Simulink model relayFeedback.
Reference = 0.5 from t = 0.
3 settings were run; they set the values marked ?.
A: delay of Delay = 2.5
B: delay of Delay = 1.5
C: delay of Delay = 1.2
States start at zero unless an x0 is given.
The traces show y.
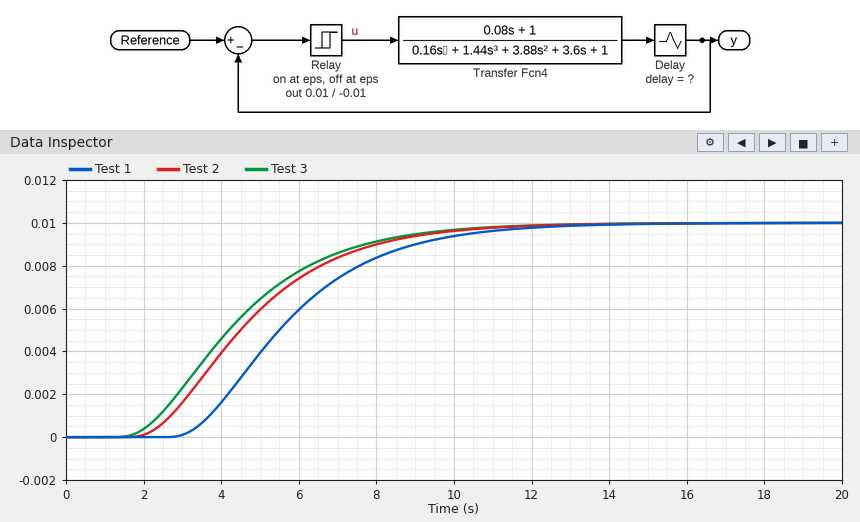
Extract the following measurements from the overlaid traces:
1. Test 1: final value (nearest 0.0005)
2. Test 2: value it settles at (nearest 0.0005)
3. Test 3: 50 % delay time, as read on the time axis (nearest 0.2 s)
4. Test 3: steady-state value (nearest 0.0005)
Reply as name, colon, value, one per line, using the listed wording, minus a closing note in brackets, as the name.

Test 1: final value: 0.0100
Test 2: value it settles at: 0.0100
Test 3: 50 % delay time, as read on the time axis: 4.2 s
Test 3: steady-state value: 0.0100
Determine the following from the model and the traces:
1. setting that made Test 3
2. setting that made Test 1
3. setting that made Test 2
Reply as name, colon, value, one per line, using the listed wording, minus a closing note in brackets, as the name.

setting that made Test 3: C
setting that made Test 1: A
setting that made Test 2: B
